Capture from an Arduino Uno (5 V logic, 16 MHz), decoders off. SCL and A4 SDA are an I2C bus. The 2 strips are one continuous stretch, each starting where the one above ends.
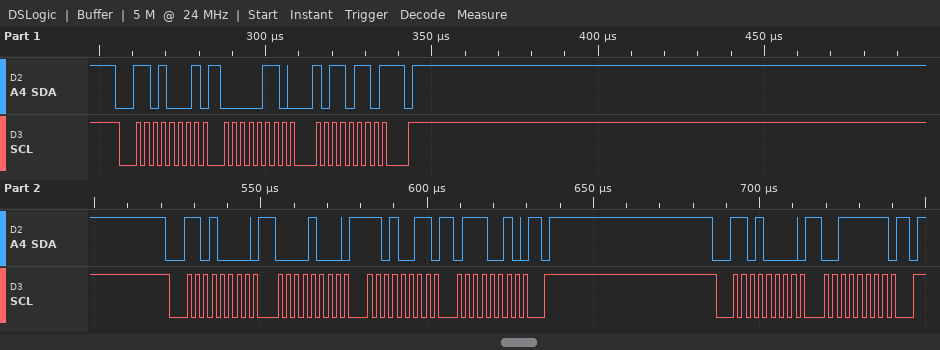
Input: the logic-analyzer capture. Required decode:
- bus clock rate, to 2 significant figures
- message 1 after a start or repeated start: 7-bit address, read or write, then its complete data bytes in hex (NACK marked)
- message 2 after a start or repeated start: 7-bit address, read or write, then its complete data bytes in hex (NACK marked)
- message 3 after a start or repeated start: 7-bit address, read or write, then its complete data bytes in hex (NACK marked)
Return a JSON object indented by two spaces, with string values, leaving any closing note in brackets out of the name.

{
  "bus clock rate, to 2 significant figures": "400 kHz",
  "message 1 after a start or repeated start: 7-bit address, read or write, then its complete data bytes in hex": "0x68 read: 06 B6 NACK",
  "message 2 after a start or repeated start: 7-bit address, read or write, then its complete data bytes in hex": "0x68 write: 08 D3 72",
  "message 3 after a start or repeated start: 7-bit address, read or write, then its complete data bytes in hex": "0x68 write: 3F"
}
